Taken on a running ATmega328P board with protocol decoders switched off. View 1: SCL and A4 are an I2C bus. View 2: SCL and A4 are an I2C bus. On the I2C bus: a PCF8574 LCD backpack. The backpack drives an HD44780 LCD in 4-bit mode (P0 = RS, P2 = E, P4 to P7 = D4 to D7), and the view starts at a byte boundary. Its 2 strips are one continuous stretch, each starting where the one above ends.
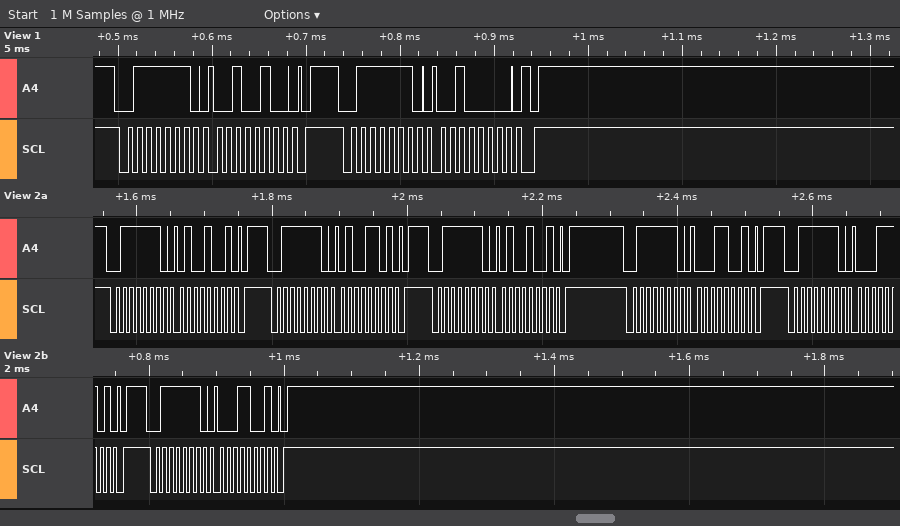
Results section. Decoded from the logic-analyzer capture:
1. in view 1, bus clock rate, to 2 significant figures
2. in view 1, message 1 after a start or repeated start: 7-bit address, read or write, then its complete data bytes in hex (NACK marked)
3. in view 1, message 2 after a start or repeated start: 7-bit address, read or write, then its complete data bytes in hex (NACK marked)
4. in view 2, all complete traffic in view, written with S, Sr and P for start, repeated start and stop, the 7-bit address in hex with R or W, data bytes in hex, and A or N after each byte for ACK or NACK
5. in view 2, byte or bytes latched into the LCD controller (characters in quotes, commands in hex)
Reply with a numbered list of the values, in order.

1. 100 kHz
2. 0x3F write: 24
3. 0x3F write: 20
4. S 3FW A 49 A P S 3FW A 4D A P S 3FW A 49 A P S 3FW A 19 A P S 3FW A 1D A P S 3FW A 19 A P
5. 'A'
